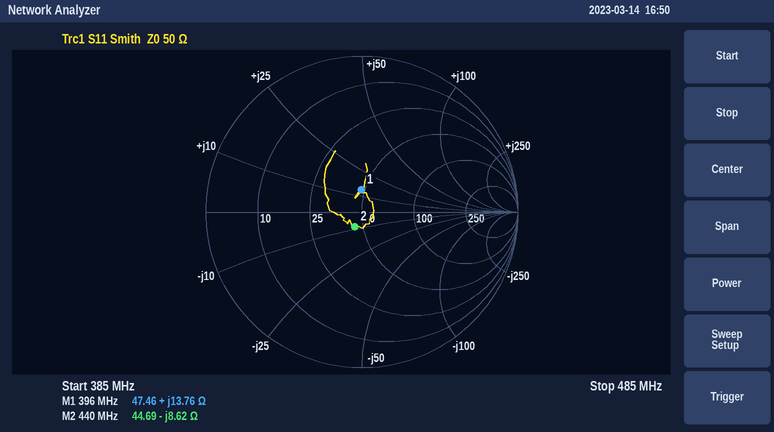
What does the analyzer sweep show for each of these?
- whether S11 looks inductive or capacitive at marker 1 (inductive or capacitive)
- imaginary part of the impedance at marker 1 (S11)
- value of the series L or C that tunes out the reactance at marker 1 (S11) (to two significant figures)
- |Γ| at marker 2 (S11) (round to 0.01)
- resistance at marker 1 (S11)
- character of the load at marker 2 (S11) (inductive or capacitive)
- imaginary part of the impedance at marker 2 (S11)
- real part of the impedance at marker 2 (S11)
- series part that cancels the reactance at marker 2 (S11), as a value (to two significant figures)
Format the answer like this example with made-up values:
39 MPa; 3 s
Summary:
inductive; +13.76 Ω; 29 pF; 0.11; 47.46 Ω; capacitive; -8.62 Ω; 44.69 Ω; 3.1 nH
